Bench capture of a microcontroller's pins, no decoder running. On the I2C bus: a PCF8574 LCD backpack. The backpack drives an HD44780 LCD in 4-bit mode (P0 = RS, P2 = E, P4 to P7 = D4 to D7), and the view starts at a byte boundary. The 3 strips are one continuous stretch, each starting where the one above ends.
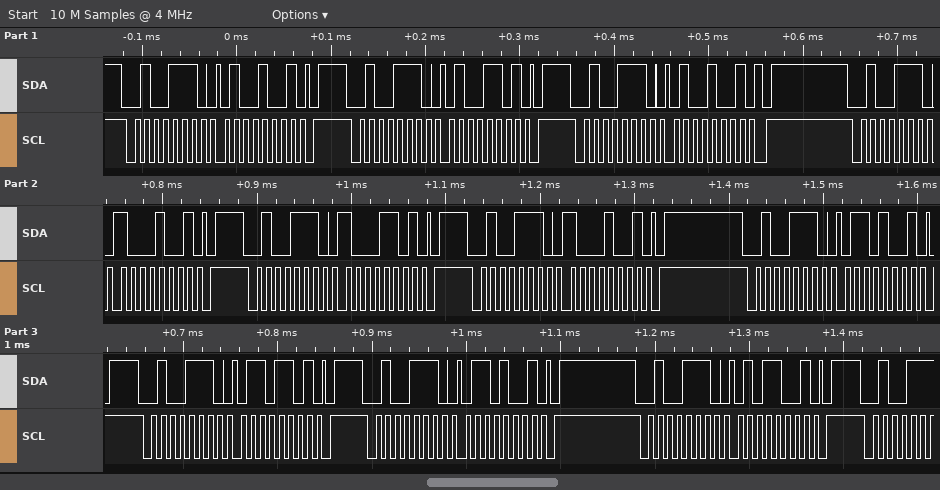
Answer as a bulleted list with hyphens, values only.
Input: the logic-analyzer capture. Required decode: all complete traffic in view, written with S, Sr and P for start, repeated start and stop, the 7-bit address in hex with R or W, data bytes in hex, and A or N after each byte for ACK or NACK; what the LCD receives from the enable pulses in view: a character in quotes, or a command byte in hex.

- S 27W A 49 A P S 27W A 4D A P S 27W A 49 A P S 27W A 89 A P S 27W A 8D A P S 27W A 89 A P S 27W A 69 A P S 27W A 6D A P S 27W A 69 A P S 27W A 59 A P
- 'H'
